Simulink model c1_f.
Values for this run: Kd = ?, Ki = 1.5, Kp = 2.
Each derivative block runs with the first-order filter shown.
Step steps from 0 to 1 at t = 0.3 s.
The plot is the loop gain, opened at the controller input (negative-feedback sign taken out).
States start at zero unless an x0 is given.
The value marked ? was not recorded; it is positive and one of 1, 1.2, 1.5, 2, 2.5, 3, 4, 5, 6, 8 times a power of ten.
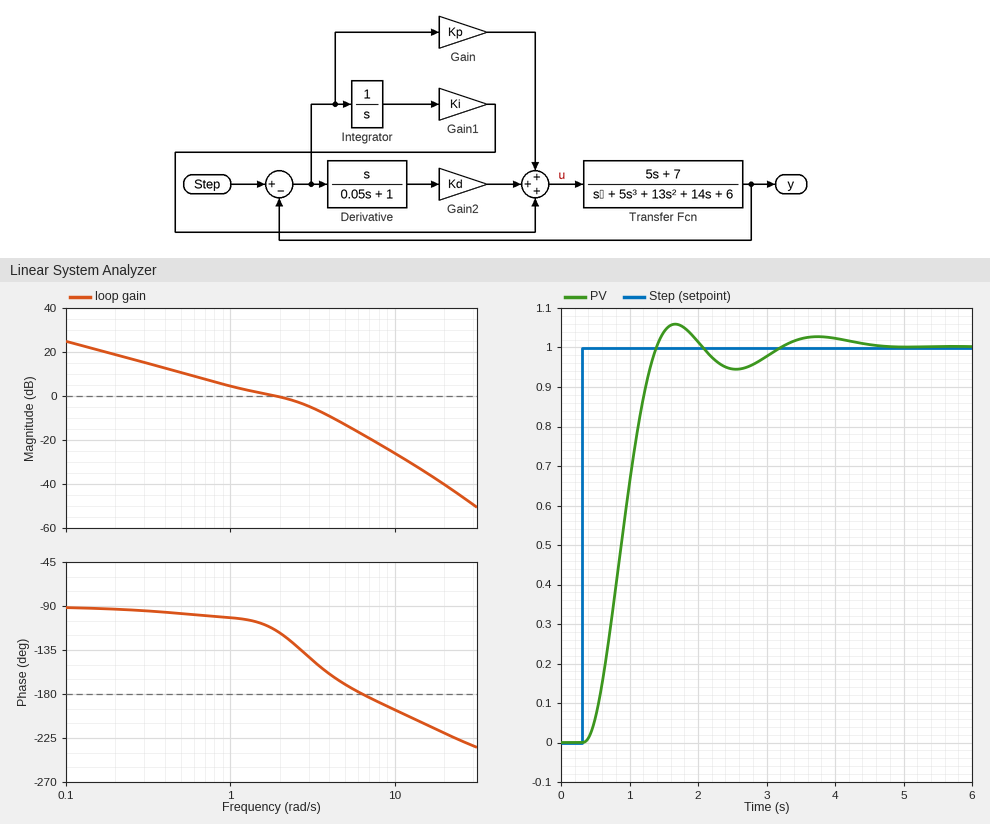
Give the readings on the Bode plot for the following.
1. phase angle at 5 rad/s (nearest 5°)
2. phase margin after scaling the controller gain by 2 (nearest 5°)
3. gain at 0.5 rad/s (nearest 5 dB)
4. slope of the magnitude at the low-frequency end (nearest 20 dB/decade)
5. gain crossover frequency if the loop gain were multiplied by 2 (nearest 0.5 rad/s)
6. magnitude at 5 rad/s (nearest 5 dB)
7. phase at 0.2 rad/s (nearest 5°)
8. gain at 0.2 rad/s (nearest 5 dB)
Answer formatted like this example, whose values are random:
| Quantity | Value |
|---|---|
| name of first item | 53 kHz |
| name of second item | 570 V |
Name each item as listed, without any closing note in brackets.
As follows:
| Quantity | Value |
|---|---|
| phase angle at 5 rad/s | -170° |
| phase margin after scaling the controller gain by 2 | 30° |
| gain at 0.5 rad/s | 10 dB |
| slope of the magnitude at the low-frequency end | -20 dB/decade |
| gain crossover frequency if the loop gain were multiplied by 2 | 3.5 rad/s |
| magnitude at 5 rad/s | -15 dB |
| phase at 0.2 rad/s | -95° |
| gain at 0.2 rad/s | 20 dB |
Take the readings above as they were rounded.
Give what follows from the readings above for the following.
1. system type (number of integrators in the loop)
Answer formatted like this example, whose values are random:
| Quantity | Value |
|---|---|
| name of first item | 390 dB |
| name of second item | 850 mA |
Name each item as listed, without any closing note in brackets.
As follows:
| Quantity | Value |
|---|---|
| system type | 1 |
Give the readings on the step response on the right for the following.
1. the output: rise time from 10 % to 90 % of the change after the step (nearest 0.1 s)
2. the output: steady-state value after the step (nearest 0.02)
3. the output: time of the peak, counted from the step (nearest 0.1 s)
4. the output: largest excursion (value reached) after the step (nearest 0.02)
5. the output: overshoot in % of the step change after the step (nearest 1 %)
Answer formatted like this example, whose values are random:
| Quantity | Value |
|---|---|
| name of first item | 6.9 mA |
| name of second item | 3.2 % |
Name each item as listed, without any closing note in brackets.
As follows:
| Quantity | Value |
|---|---|
| the output: rise time from 10 % to 90 % of the change after the step | 0.7 s |
| the output: steady-state value after the step | 1.00 |
| the output: time of the peak, counted from the step | 1.4 s |
| the output: largest excursion (value reached) after the step | 1.06 |
| the output: overshoot in % of the step change after the step | 6 % |
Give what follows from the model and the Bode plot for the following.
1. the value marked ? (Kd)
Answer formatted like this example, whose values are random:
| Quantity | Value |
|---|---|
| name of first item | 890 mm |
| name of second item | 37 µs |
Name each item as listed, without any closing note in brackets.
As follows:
| Quantity | Value |
|---|---|
| the value marked ? | 1 |
